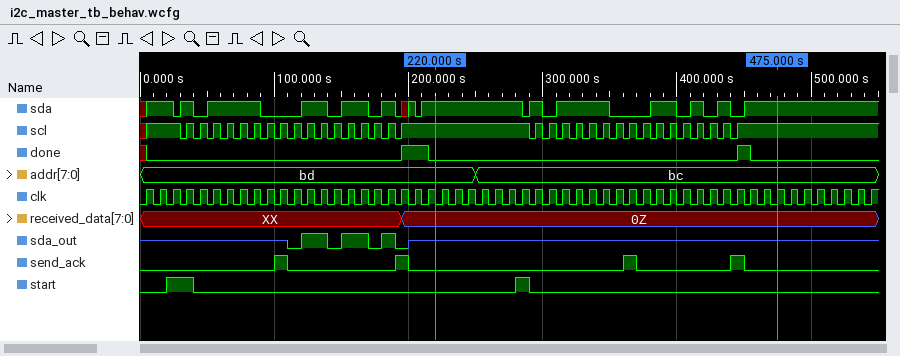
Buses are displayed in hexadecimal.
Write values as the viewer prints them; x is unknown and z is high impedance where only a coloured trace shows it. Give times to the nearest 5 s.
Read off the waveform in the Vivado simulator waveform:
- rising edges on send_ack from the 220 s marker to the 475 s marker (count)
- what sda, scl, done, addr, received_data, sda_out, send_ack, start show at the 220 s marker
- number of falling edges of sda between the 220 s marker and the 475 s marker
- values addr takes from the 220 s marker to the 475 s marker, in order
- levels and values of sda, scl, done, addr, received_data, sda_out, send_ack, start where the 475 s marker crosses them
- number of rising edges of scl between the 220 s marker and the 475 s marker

2
sda=1, scl=1, done=0, addr=bd, received_data=0Z, sda_out=z, send_ack=0, start=0
6
bd, bc
sda=1, scl=1, done=0, addr=bc, received_data=0Z, sda_out=z, send_ack=0, start=0
16
